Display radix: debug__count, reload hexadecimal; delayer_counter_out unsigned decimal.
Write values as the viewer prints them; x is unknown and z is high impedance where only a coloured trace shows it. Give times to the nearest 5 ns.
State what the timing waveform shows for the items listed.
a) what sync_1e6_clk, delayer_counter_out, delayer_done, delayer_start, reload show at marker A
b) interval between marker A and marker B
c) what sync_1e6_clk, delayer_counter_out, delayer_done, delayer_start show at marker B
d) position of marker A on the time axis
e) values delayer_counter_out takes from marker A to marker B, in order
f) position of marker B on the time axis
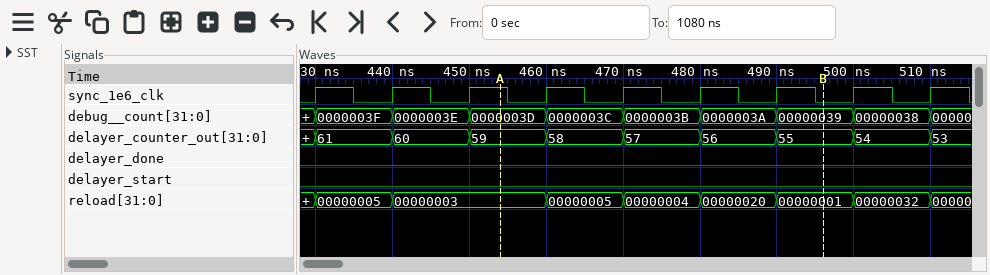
sync_1e6_clk=1, delayer_counter_out=59, delayer_done=0, delayer_start=0, reload=00000003
40 ns
sync_1e6_clk=0, delayer_counter_out=55, delayer_done=0, delayer_start=0
455 ns
59, 58, 57, 56, 55
495 ns
